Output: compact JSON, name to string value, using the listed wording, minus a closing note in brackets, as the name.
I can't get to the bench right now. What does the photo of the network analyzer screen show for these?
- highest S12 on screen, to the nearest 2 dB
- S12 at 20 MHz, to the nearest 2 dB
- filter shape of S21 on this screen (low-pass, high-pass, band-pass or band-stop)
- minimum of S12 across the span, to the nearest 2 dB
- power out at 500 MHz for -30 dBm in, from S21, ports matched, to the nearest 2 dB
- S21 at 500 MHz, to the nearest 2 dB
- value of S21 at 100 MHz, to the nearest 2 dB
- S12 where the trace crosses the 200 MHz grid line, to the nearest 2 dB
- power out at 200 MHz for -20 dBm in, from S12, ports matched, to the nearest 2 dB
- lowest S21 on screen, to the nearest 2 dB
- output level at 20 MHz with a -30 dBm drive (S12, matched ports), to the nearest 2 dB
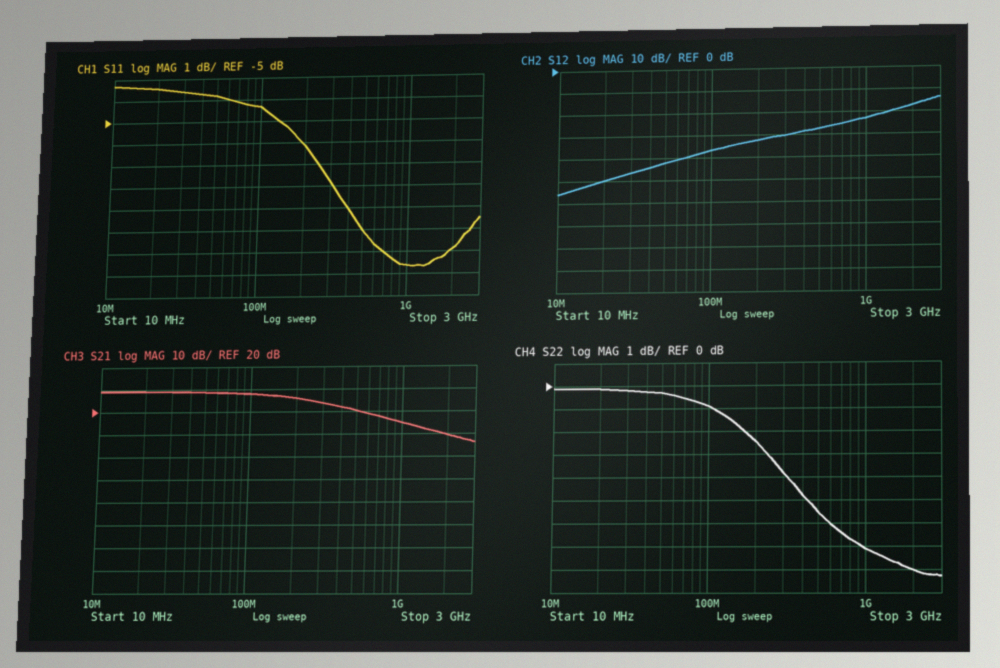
{"highest S12 on screen, to the nearest 2 dB": "-14 dB", "S12 at 20 MHz, to the nearest 2 dB": "-50 dB", "filter shape of S21 on this screen": "low-pass", "minimum of S12 across the span, to the nearest 2 dB": "-56 dB", "power out at 500 MHz for -30 dBm in, from S21, ports matched, to the nearest 2 dB": "-10 dBm", "S21 at 500 MHz, to the nearest 2 dB": "20 dB", "value of S21 at 100 MHz, to the nearest 2 dB": "28 dB", "S12 where the trace crosses the 200 MHz grid line, to the nearest 2 dB": "-32 dB", "power out at 200 MHz for -20 dBm in, from S12, ports matched, to the nearest 2 dB": "-52 dBm", "lowest S21 on screen, to the nearest 2 dB": "6 dB", "output level at 20 MHz with a -30 dBm drive (S12, matched ports), to the nearest 2 dB": "-80 dBm"}
